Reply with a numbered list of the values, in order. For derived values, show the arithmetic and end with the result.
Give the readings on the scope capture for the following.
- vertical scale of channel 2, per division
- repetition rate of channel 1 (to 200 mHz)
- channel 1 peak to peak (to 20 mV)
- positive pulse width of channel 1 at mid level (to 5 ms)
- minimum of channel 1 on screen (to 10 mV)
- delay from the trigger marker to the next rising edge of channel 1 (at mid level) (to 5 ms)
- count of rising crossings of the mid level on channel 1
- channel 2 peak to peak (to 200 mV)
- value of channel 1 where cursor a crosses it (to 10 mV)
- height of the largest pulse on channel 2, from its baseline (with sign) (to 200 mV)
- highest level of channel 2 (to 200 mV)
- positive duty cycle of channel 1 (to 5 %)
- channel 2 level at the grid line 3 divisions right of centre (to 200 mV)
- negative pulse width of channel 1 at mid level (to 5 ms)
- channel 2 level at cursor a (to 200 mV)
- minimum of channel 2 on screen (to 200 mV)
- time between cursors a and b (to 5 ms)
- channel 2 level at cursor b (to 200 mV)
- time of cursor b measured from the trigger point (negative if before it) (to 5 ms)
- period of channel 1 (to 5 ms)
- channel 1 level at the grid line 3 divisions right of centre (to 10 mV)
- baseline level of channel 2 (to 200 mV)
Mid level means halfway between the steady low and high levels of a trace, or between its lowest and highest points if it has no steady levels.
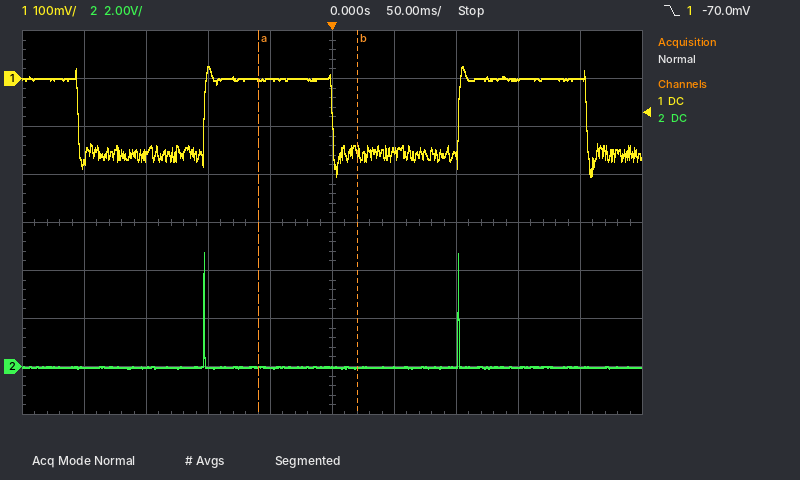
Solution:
1. 2 V
2. 1 / 205 ms ≈ 4.88 Hz, so 4.8 Hz to the nearest 200 mHz
3. 220 mV
4. 105 ms
5. -200 mV
6. 100 ms
7. 2
8. 4.8 V − (0.0 V) = 4.8 V
9. 0 mV
10. 4.8 V − (0.0 V) = +4.8 V
11. 4.8 V
12. 105 ms / 205 ms ≈ 51.2 %, so 50 % to the nearest 5 %
13. 0.0 V
14. 100 ms
15. 0.0 V
16. 0.0 V
17. 80 ms
18. 0.0 V
19. +20 ms
20. 205 ms
21. 0 mV
22. 0.0 V
